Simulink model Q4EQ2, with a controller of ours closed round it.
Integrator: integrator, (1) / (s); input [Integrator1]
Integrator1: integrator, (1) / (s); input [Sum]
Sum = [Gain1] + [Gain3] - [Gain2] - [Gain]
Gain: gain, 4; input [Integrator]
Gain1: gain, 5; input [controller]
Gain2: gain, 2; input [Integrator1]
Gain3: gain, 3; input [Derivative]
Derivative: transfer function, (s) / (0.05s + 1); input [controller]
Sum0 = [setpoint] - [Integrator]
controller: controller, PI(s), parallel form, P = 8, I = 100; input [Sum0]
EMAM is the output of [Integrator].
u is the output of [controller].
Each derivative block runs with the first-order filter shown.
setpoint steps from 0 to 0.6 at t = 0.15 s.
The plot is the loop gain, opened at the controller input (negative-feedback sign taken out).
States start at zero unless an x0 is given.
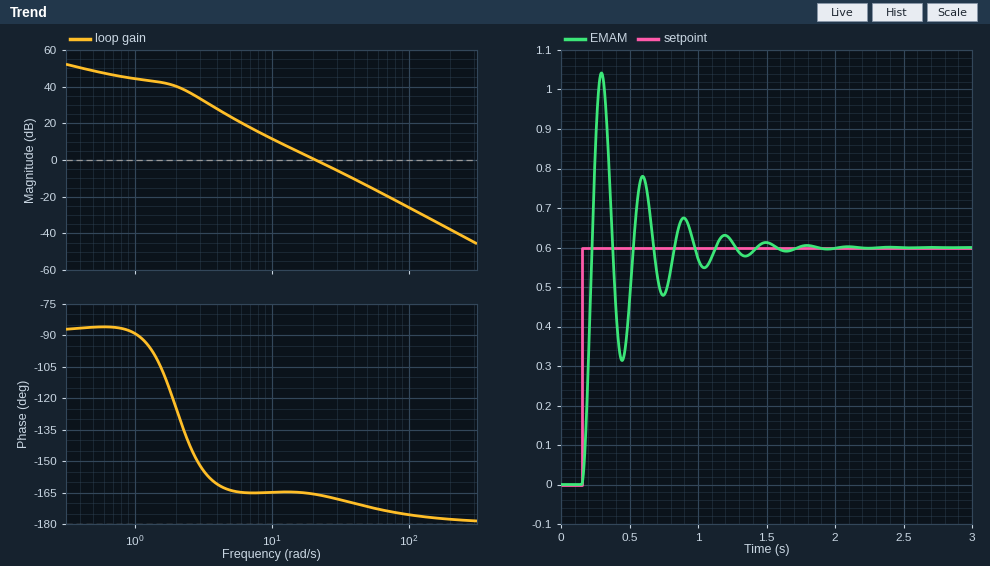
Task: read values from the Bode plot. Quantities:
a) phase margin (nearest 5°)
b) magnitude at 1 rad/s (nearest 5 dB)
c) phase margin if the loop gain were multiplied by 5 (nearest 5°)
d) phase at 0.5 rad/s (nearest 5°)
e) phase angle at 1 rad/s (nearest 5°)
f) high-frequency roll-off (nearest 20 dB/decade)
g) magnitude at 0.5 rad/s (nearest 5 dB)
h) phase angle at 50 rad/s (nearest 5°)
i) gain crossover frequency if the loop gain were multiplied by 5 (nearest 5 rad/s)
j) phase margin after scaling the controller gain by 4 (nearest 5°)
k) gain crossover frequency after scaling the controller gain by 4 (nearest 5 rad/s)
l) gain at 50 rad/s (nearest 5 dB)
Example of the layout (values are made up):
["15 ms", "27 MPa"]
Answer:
["15°", "45 dB", "10°", "-85°", "-90°", "-40 dB/decade", "50 dB", "-170°", "50 rad/s", "10°", "45 rad/s", "-15 dB"]
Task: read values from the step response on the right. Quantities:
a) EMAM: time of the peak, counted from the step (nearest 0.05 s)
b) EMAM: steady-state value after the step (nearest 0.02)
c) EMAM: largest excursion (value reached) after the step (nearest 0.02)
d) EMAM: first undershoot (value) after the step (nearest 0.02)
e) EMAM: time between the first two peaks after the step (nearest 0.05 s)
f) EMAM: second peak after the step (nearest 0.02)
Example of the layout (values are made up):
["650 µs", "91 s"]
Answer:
["0.15 s", "0.60", "1.04", "0.32", "0.30 s", "0.78"]
